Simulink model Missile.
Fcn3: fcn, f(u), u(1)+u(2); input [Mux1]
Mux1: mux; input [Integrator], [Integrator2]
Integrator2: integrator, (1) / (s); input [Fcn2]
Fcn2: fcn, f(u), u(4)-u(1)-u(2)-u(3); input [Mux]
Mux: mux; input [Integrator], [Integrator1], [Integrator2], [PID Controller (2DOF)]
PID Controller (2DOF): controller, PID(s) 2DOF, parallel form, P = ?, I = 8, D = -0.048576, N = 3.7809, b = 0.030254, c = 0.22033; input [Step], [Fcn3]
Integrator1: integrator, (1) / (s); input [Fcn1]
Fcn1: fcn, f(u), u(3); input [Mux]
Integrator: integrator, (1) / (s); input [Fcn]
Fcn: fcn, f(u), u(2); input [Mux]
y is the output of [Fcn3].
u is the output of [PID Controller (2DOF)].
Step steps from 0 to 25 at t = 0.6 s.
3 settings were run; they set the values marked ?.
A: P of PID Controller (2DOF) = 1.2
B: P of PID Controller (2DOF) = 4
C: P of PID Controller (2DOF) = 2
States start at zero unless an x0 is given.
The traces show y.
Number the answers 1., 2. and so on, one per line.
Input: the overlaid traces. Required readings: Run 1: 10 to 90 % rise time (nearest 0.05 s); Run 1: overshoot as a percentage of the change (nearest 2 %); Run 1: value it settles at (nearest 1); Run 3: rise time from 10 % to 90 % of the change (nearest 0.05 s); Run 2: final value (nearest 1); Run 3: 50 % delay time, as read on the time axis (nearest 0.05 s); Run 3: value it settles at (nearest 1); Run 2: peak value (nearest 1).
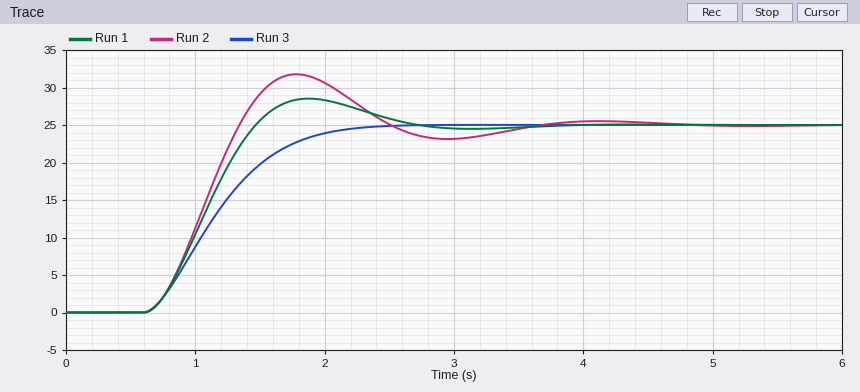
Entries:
1. 0.60 s
2. 14 %
3. 25
4. 1.00 s
5. 25
6. 1.15 s
7. 25
8. 32
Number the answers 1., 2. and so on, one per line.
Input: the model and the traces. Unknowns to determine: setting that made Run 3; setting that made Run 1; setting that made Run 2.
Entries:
1. B
2. C
3. A
